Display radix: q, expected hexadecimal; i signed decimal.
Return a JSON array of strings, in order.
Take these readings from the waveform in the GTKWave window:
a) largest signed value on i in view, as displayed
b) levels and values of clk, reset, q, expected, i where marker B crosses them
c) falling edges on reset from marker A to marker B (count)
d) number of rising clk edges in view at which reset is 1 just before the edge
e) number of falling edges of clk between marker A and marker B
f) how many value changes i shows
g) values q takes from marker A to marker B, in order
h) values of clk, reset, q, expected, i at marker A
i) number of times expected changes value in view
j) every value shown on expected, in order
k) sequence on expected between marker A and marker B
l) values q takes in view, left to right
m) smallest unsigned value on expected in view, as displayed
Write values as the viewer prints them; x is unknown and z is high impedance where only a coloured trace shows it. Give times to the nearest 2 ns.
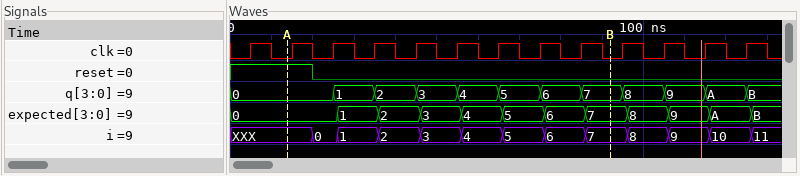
["11", "clk=0, reset=0, q=7, expected=7, i=7", "1", "2", "8", "12", "0, 1, 2, 3, 4, 5, 6, 7", "clk=0, reset=1, q=0, expected=0, i=XXX", "11", "0, 1, 2, 3, 4, 5, 6, 7, 8, 9, A, B", "0, 1, 2, 3, 4, 5, 6, 7", "0, 1, 2, 3, 4, 5, 6, 7, 8, 9, A, B", "0"]
